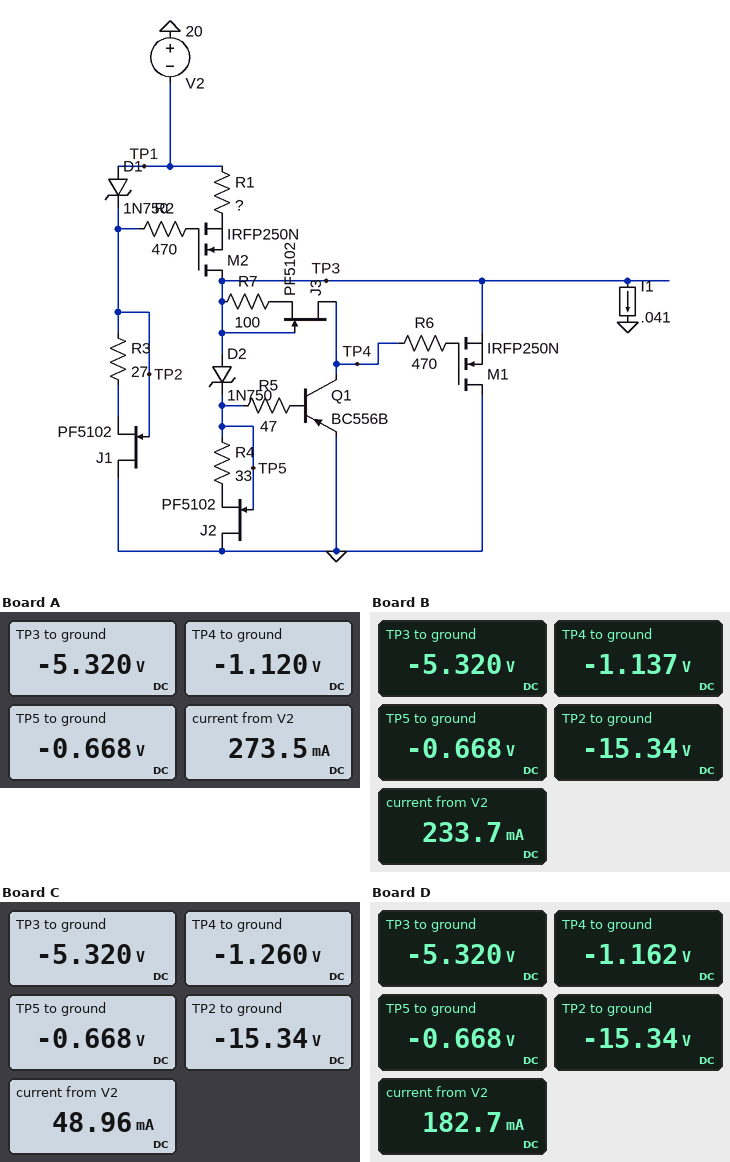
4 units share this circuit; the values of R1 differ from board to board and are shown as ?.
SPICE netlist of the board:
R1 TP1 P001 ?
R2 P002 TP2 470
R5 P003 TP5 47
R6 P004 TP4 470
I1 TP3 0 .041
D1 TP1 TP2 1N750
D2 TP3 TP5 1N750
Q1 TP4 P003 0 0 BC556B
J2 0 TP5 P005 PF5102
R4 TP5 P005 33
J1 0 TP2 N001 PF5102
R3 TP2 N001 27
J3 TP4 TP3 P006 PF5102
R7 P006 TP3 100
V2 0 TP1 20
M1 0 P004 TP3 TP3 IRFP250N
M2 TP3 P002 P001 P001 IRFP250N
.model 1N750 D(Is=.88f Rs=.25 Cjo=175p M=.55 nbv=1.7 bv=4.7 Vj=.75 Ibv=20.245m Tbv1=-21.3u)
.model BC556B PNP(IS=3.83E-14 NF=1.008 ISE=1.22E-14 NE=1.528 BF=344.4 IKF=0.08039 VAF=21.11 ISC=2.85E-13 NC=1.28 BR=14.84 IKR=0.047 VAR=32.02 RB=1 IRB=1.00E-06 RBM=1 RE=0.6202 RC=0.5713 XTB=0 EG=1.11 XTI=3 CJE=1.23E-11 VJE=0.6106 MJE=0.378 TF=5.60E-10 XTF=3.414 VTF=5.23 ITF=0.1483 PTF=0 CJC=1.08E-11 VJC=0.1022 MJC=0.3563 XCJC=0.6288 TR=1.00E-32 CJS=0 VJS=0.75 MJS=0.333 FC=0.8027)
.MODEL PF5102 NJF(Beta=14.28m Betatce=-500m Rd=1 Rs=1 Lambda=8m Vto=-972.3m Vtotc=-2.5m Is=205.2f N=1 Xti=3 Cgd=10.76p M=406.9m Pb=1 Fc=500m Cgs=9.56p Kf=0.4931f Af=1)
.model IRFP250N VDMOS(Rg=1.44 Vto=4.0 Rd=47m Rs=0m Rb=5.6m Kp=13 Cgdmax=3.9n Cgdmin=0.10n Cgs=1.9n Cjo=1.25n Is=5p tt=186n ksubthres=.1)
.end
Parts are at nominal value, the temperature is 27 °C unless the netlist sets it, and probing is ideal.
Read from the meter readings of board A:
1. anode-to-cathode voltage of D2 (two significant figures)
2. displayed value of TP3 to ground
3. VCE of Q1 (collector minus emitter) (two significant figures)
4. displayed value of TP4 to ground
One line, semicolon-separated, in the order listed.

-4.7 V; -5.320 V; -1.1 V; -1.120 V
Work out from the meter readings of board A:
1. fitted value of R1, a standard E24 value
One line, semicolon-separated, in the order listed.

1.8 Ω
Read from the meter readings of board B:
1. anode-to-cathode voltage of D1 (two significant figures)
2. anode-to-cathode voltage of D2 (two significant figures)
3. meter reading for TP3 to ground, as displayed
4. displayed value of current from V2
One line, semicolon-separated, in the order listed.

-4.7 V; -4.7 V; -5.320 V; 233.7 mA
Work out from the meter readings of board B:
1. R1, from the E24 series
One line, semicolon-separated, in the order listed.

2.2 Ω
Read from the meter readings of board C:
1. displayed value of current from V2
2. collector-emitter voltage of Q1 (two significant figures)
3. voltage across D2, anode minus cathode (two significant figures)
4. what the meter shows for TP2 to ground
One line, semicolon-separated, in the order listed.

48.96 mA; -1.3 V; -4.7 V; -15.34 V
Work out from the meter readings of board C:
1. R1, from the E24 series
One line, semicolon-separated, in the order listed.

16 Ω
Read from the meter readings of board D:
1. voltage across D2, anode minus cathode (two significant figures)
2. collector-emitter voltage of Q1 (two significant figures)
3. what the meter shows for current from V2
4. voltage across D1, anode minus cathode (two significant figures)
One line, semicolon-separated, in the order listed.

-4.7 V; -1.2 V; 182.7 mA; -4.7 V
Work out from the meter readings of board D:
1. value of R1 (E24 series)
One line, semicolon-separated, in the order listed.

3 Ω
